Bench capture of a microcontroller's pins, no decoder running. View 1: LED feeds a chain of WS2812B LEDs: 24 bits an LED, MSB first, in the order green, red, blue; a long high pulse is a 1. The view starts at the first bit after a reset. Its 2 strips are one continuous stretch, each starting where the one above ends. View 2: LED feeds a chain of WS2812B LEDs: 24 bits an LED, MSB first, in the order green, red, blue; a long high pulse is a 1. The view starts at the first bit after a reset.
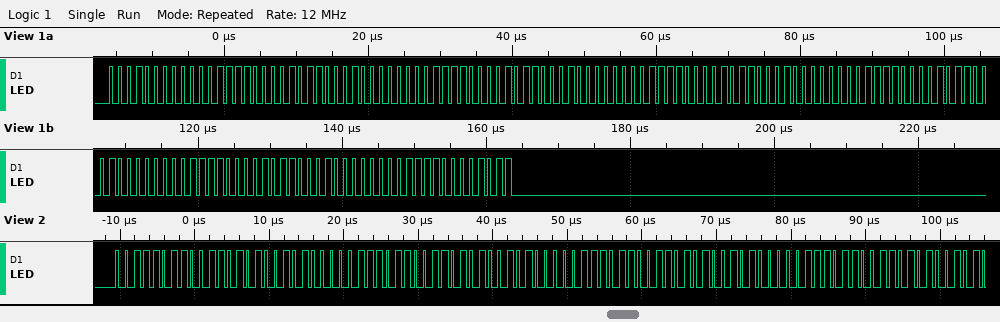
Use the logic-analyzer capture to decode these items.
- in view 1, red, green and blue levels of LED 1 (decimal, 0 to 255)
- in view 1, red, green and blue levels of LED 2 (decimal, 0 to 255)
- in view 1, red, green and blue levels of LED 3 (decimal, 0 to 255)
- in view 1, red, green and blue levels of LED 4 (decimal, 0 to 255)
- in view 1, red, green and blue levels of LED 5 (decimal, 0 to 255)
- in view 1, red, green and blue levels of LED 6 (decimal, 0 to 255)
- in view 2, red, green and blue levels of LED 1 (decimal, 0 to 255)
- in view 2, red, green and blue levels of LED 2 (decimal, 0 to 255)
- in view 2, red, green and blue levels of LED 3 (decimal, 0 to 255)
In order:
15, 16, 11
15, 16, 11
15, 16, 11
15, 16, 11
15, 16, 11
15, 16, 11
53, 59, 40
53, 59, 40
53, 59, 40
